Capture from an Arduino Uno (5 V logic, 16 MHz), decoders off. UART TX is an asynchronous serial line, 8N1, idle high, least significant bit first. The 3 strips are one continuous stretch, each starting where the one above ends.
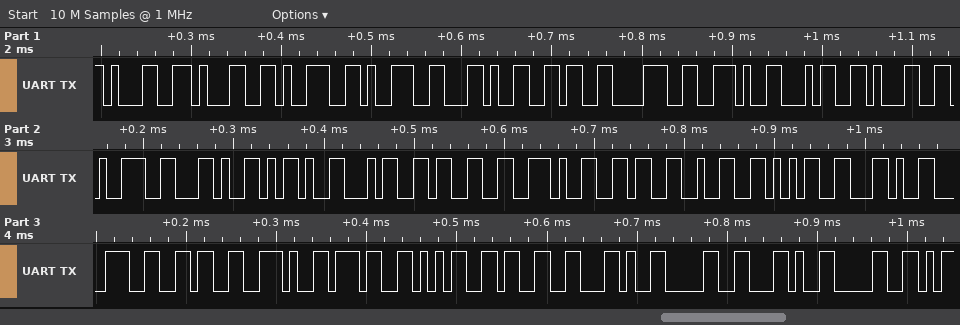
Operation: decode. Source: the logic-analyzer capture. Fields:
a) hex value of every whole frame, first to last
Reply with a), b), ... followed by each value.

a) 31 31 39 39 2C 36 38 2E 34 31 39 2C 2D 34 33 2E 36 32 35 2C 38 36 2E 37 35 33 2C 30 2C 30
